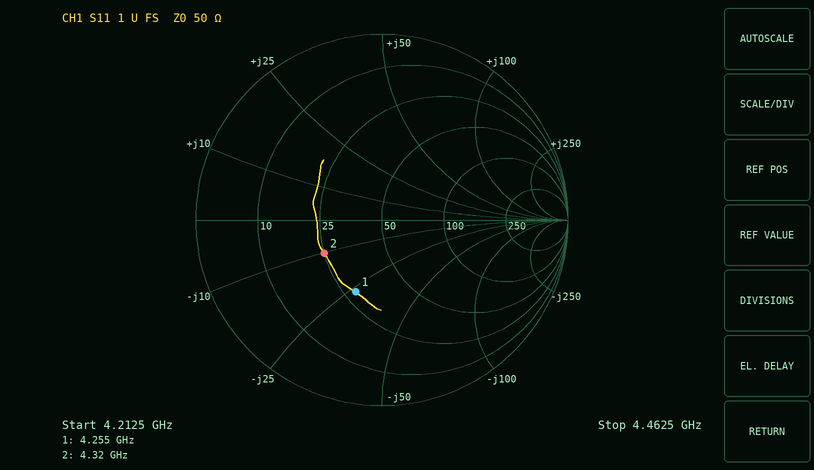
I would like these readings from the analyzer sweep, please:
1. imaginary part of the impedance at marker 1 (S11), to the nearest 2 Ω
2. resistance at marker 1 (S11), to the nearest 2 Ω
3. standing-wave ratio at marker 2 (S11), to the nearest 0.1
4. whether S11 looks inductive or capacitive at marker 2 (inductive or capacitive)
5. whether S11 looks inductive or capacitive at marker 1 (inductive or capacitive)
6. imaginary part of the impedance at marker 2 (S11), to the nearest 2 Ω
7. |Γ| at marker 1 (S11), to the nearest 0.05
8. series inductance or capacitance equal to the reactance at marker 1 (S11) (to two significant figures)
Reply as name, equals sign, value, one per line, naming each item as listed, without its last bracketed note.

imaginary part of the impedance at marker 1 (S11), to the nearest 2 Ω = -26 Ω
resistance at marker 1 (S11), to the nearest 2 Ω = 28 Ω
standing-wave ratio at marker 2 (S11), to the nearest 0.1 = 2.1
whether S11 looks inductive or capacitive at marker 2 = capacitive
whether S11 looks inductive or capacitive at marker 1 = capacitive
imaginary part of the impedance at marker 2 (S11), to the nearest 2 Ω = -10 Ω
|Γ| at marker 1 (S11), to the nearest 0.05 = 0.40
series inductance or capacitance equal to the reactance at marker 1 (S11) = 1.4 pF
